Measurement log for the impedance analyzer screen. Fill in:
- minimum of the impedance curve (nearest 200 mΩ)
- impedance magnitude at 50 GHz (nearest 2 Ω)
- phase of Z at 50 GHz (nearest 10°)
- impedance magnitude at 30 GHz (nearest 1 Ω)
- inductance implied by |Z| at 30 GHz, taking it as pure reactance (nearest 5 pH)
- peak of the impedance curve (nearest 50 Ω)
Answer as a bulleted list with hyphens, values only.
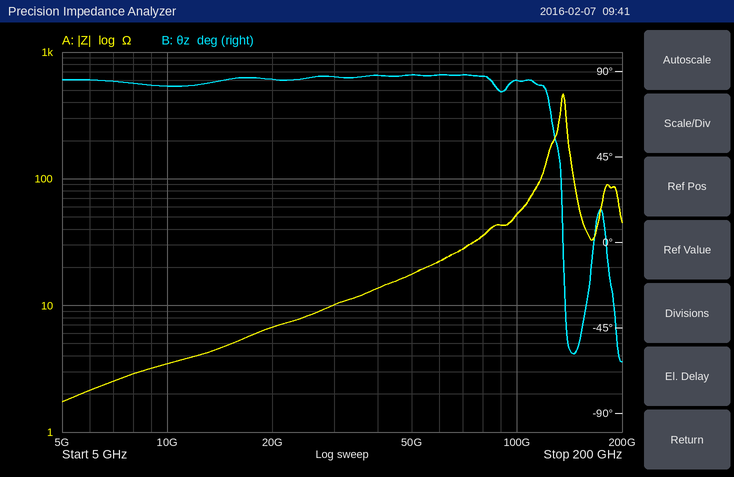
- 1.8 Ω
- 18 Ω
- 90°
- 10 Ω
- 55 pH
- 450 Ω
